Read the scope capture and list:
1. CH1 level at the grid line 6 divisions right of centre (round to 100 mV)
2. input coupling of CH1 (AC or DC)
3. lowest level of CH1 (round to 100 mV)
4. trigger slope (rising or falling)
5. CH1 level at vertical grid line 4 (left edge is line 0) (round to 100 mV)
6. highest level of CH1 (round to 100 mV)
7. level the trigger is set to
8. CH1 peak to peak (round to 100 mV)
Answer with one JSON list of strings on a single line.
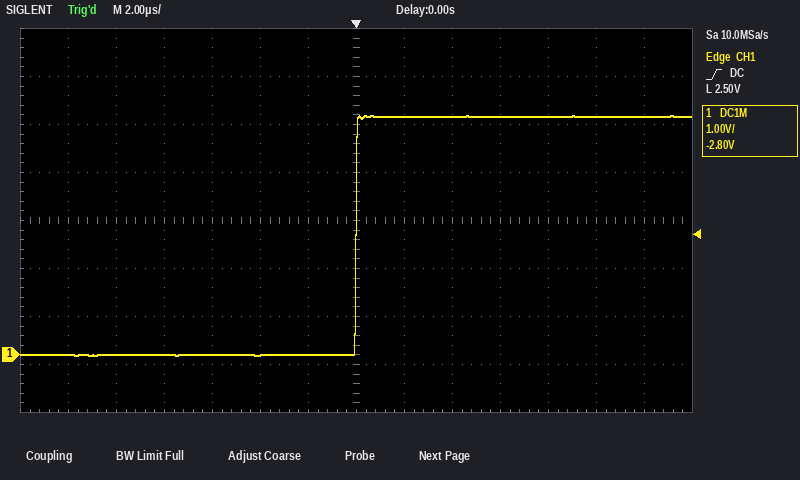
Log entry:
["5.0 V", "DC", "0.0 V", "rising", "0.0 V", "5.0 V", "2.50 V", "5.0 V"]
